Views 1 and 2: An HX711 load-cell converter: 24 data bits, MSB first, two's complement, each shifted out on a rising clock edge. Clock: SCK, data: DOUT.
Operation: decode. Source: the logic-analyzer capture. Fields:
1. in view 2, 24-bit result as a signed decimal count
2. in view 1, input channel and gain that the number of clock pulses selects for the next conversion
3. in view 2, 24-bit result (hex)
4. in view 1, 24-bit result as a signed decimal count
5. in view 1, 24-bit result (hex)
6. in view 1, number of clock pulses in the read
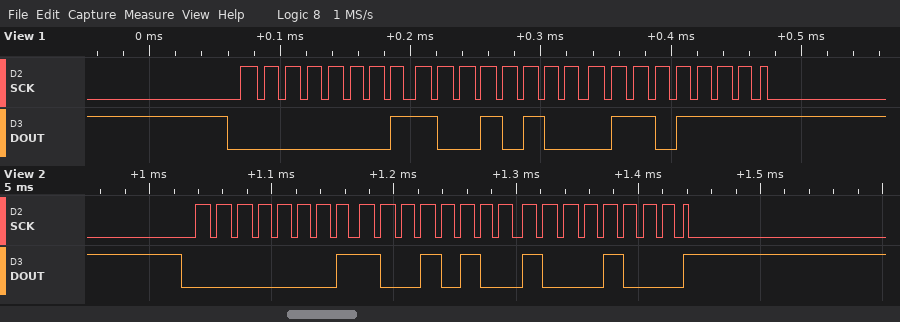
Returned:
103560
channel A, gain 128
0x019488
103535
0x01946F
25
